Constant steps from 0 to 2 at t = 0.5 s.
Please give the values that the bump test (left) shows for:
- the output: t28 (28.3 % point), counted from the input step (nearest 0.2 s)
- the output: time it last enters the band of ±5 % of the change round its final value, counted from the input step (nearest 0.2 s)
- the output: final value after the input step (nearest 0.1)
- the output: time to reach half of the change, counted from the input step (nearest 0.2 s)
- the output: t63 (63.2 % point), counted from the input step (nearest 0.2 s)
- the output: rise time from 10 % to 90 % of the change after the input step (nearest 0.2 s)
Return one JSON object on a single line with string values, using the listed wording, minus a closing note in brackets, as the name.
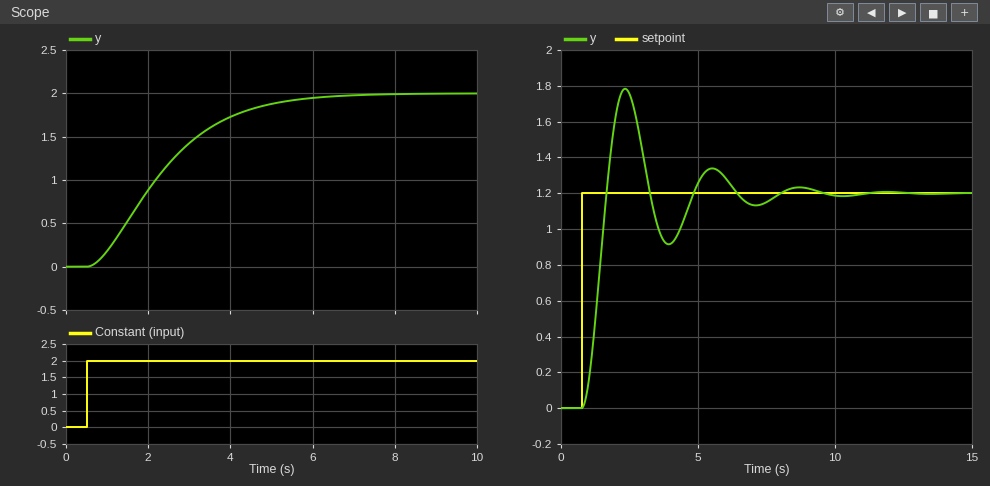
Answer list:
{"the output: t28 (28.3 % point), counted from the input step": "1.0 s", "the output: time it last enters the band of ±5 % of the change round its final value, counted from the input step": "4.8 s", "the output: final value after the input step": "2.0", "the output: time to reach half of the change, counted from the input step": "1.6 s", "the output: t63 (63.2 % point), counted from the input step": "2.2 s", "the output: rise time from 10 % to 90 % of the change after the input step": "3.4 s"}
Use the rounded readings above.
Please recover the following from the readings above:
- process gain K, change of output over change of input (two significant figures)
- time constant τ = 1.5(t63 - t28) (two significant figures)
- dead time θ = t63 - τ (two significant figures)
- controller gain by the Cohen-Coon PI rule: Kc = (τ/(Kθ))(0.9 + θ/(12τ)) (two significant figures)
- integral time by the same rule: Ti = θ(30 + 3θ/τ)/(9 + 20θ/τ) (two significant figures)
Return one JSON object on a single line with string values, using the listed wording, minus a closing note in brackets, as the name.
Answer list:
{"process gain K, change of output over change of input": "1.0", "time constant τ = 1.5(t63 - t28)": "1.8 s", "dead time θ = t63 - τ": "0.40 s", "controller gain by the Cohen-Coon PI rule: Kc = (τ/(Kθ))(0.9 + θ/(12τ))": "4.1", "integral time by the same rule: Ti = θ(30 + 3θ/τ)/(9 + 20θ/τ)": "0.91 s"}
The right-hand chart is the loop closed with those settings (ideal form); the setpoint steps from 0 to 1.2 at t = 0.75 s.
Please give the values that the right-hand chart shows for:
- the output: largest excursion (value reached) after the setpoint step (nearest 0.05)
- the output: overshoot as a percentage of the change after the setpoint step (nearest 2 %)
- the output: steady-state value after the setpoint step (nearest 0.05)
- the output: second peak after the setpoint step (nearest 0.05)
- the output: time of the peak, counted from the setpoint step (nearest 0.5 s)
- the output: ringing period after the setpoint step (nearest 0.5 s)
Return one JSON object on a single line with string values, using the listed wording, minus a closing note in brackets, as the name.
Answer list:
{"the output: largest excursion (value reached) after the setpoint step": "1.80", "the output: overshoot as a percentage of the change after the setpoint step": "48 %", "the output: steady-state value after the setpoint step": "1.20", "the output: second peak after the setpoint step": "1.35", "the output: time of the peak, counted from the setpoint step": "1.5 s", "the output: ringing period after the setpoint step": "3.0 s"}
